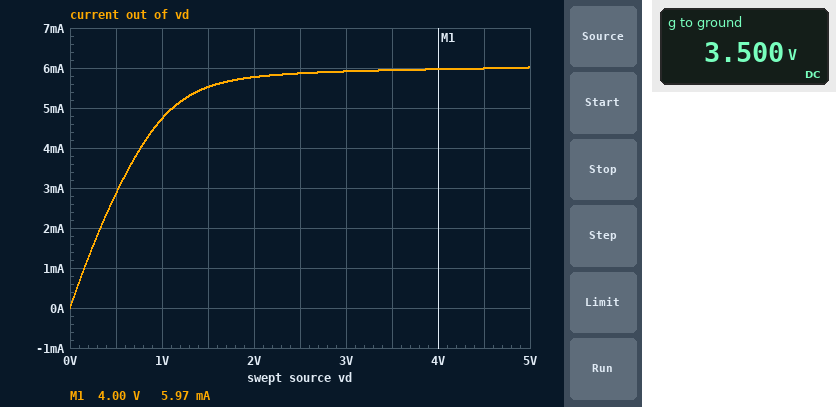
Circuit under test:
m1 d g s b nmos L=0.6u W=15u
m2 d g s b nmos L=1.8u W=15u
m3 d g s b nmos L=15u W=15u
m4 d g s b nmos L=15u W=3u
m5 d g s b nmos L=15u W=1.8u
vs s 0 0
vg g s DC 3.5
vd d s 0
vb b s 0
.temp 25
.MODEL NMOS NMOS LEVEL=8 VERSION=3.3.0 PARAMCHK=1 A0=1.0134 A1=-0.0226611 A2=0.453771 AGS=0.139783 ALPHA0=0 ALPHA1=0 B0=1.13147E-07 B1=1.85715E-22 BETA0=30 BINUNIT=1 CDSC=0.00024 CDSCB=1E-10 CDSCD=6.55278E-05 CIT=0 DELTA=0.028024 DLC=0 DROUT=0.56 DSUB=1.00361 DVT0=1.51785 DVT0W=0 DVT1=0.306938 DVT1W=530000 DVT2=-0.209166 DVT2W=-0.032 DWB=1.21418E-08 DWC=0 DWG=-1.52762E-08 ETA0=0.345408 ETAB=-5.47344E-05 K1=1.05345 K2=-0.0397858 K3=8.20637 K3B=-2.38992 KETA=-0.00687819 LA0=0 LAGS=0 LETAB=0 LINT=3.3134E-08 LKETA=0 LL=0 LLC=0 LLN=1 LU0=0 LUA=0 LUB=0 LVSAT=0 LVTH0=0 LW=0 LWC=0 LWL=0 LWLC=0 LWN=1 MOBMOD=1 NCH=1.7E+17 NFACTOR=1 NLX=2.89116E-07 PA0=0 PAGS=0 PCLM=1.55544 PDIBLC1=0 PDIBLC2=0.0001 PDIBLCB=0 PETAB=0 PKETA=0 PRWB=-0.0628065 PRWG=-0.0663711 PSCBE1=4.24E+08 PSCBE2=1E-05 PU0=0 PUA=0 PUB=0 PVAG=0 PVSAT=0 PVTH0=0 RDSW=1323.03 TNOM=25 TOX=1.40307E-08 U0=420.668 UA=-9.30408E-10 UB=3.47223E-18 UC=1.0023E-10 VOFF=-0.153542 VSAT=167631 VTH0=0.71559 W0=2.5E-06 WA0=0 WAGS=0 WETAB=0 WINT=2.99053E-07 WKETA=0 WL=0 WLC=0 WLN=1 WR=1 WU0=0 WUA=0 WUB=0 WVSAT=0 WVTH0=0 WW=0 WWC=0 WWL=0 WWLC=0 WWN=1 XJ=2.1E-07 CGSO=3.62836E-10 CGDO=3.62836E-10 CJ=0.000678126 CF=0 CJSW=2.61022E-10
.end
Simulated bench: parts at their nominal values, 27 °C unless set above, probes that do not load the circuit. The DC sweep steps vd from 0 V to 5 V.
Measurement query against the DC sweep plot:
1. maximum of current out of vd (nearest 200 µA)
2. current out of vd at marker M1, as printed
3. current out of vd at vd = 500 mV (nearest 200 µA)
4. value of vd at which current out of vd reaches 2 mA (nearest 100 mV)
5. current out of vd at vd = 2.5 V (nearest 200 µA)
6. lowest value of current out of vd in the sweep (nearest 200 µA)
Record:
6.0 mA
5.97 mA
2.8 mA
300 mV
5.8 mA
0 A
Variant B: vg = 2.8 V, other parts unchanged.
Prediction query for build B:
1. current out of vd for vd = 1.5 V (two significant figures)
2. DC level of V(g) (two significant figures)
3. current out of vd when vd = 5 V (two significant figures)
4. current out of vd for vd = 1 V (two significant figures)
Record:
3.7 mA
2.8 V
3.9 mA
3.3 mA
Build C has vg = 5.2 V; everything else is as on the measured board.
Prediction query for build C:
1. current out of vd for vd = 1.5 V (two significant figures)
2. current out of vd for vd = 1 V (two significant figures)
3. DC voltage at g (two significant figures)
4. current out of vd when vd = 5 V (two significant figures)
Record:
9.3 mA
7.2 mA
5.2 V
11 mA
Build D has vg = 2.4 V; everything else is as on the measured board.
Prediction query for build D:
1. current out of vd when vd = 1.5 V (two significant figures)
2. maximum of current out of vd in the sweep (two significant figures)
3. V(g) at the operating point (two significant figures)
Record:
2.6 mA
2.8 mA
2.4 V
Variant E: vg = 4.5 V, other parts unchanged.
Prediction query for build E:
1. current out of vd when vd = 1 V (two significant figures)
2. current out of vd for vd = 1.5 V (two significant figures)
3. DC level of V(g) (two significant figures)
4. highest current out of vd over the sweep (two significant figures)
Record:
6.3 mA
7.9 mA
4.5 V
9.2 mA
